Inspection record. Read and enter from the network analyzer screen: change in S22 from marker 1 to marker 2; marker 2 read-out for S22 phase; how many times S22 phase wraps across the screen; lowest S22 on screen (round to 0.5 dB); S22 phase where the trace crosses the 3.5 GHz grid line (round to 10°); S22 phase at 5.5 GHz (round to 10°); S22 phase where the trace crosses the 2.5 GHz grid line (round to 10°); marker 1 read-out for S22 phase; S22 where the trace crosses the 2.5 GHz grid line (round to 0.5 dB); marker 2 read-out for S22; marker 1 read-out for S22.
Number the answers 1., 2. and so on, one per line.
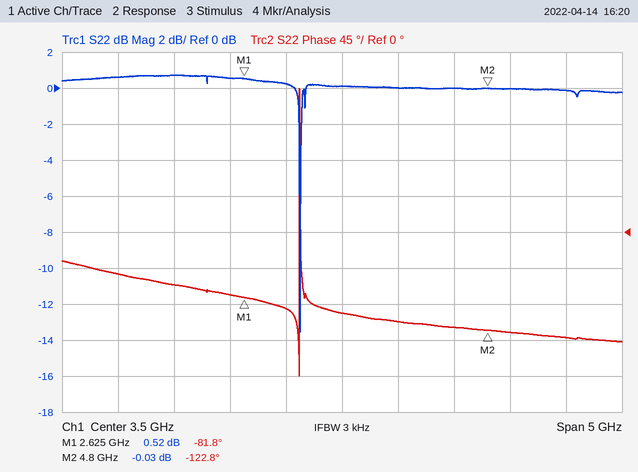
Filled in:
1. -0.55 dB
2. -122.8°
3. 1
4. -13.5 dB
5. -100°
6. -130°
7. -80°
8. -81.8°
9. 0.5 dB
10. -0.03 dB
11. 0.52 dB
